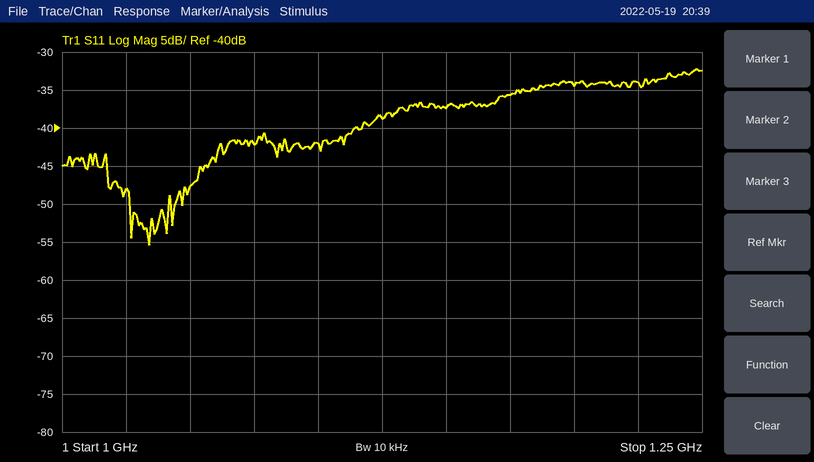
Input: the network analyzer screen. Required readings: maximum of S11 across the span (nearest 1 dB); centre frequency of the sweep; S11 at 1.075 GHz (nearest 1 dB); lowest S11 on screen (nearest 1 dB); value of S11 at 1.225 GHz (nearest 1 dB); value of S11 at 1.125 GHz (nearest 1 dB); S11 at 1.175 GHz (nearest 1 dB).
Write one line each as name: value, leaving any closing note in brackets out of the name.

maximum of S11 across the span: -32 dB
centre frequency of the sweep: 1.125 GHz
S11 at 1.075 GHz: -42 dB
lowest S11 on screen: -55 dB
value of S11 at 1.225 GHz: -34 dB
value of S11 at 1.125 GHz: -39 dB
S11 at 1.175 GHz: -36 dB
